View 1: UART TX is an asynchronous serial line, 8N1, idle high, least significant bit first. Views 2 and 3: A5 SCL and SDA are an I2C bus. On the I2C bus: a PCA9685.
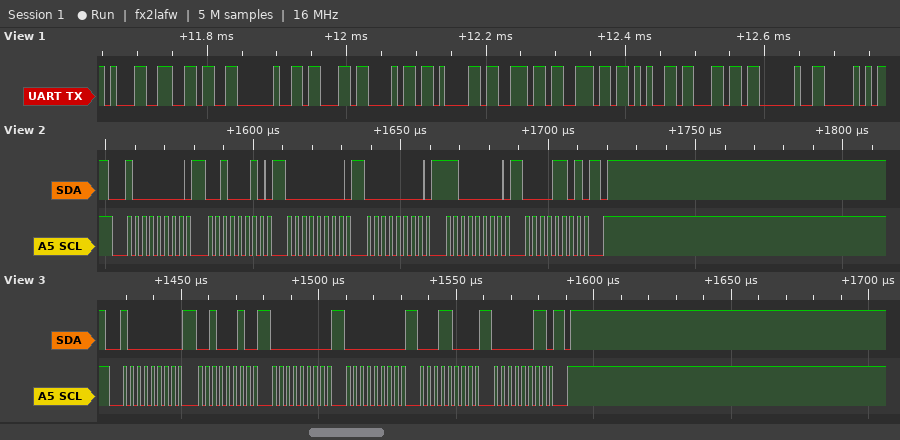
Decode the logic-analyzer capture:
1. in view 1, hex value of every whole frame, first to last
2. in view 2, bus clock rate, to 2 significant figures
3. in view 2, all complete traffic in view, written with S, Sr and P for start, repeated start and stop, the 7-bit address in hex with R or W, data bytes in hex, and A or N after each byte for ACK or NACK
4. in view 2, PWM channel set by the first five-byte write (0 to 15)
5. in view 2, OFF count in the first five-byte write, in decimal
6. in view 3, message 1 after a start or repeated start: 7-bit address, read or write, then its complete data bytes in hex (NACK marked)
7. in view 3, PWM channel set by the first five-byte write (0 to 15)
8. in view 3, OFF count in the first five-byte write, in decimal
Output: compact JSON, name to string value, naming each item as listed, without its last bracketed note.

{"in view 1, hex value of every whole frame, first to last": "31 36 20 63 68 61 6E 6E 65 6C 20 50", "in view 2, bus clock rate, to 2 significant figures": "400 kHz", "in view 2, all complete traffic in view, written with S, Sr and P for start, repeated start and stop, the 7-bit address in hex with R or W, data bytes in hex, and A or N after each byte for ACK or NACK": "S 40W A 22 A 00 A 00 A C0 A 0D A P", "in view 2, PWM channel set by the first five-byte write": "7", "in view 2, OFF count in the first five-byte write, in decimal": "3520", "in view 3, message 1 after a start or repeated start: 7-bit address, read or write, then its complete data bytes in hex": "0x40 write: 22 00 00 18 03", "in view 3, PWM channel set by the first five-byte write": "7", "in view 3, OFF count in the first five-byte write, in decimal": "792"}
